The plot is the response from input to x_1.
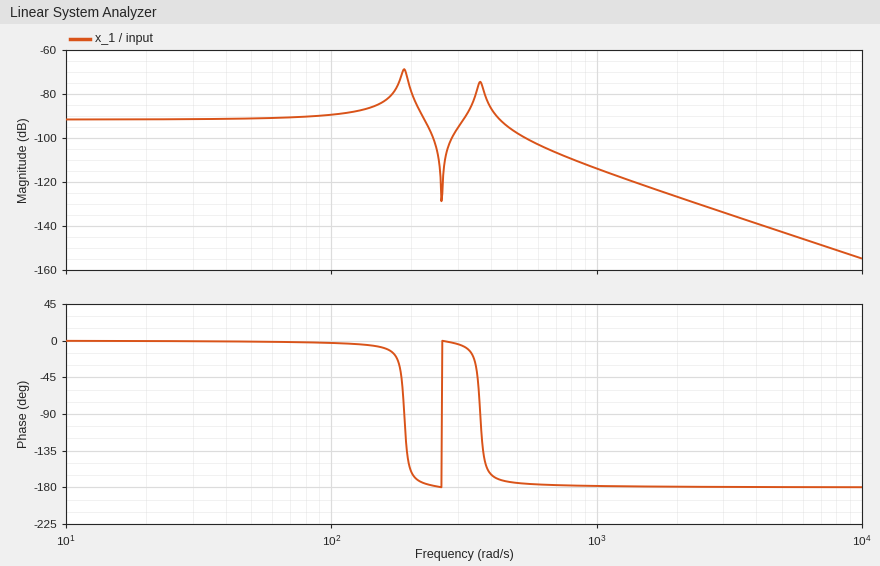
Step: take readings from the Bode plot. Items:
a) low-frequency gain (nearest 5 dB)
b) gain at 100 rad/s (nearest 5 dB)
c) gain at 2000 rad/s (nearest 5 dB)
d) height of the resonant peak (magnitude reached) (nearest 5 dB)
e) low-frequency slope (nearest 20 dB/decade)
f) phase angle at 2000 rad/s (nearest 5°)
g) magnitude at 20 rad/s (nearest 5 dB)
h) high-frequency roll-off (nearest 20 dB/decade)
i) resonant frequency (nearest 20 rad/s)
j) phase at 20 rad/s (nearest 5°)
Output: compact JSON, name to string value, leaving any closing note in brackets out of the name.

{"low-frequency gain": "-90 dB", "gain at 100 rad/s": "-90 dB", "gain at 2000 rad/s": "-125 dB", "height of the resonant peak (magnitude reached)": "-70 dB", "low-frequency slope": "0 dB/decade", "phase angle at 2000 rad/s": "-180°", "magnitude at 20 rad/s": "-90 dB", "high-frequency roll-off": "-40 dB/decade", "resonant frequency": "180 rad/s", "phase at 20 rad/s": "0°"}
